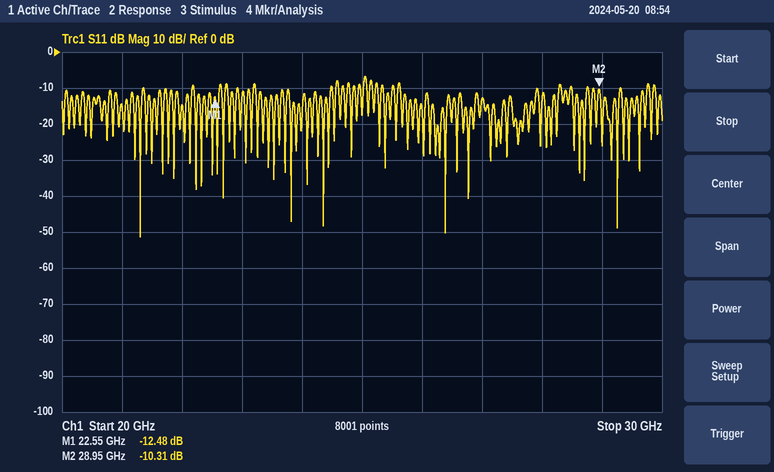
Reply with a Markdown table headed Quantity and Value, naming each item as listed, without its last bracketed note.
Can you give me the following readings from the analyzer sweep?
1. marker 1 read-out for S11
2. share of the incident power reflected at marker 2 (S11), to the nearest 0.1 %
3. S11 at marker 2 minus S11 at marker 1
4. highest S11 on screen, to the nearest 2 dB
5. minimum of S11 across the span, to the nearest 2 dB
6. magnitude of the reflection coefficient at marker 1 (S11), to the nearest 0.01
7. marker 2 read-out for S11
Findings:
| Quantity | Value |
|---|---|
| marker 1 read-out for S11 | -12.48 dB |
| share of the incident power reflected at marker 2 (S11), to the nearest 0.1 % | 9.3 % |
| S11 at marker 2 minus S11 at marker 1 | 2.17 dB |
| highest S11 on screen, to the nearest 2 dB | -6 dB |
| minimum of S11 across the span, to the nearest 2 dB | -52 dB |
| magnitude of the reflection coefficient at marker 1 (S11), to the nearest 0.01 | 0.24 |
| marker 2 read-out for S11 | -10.31 dB |
